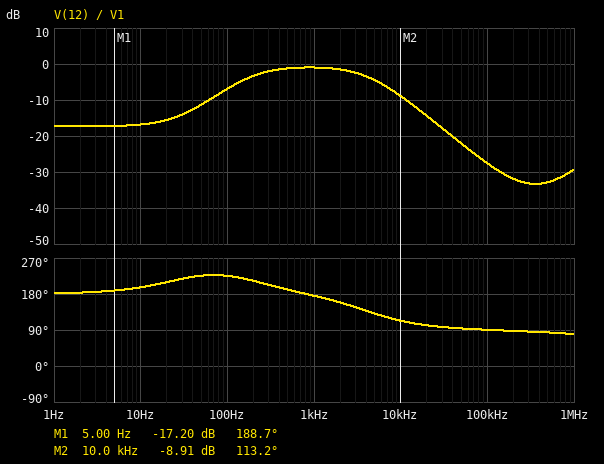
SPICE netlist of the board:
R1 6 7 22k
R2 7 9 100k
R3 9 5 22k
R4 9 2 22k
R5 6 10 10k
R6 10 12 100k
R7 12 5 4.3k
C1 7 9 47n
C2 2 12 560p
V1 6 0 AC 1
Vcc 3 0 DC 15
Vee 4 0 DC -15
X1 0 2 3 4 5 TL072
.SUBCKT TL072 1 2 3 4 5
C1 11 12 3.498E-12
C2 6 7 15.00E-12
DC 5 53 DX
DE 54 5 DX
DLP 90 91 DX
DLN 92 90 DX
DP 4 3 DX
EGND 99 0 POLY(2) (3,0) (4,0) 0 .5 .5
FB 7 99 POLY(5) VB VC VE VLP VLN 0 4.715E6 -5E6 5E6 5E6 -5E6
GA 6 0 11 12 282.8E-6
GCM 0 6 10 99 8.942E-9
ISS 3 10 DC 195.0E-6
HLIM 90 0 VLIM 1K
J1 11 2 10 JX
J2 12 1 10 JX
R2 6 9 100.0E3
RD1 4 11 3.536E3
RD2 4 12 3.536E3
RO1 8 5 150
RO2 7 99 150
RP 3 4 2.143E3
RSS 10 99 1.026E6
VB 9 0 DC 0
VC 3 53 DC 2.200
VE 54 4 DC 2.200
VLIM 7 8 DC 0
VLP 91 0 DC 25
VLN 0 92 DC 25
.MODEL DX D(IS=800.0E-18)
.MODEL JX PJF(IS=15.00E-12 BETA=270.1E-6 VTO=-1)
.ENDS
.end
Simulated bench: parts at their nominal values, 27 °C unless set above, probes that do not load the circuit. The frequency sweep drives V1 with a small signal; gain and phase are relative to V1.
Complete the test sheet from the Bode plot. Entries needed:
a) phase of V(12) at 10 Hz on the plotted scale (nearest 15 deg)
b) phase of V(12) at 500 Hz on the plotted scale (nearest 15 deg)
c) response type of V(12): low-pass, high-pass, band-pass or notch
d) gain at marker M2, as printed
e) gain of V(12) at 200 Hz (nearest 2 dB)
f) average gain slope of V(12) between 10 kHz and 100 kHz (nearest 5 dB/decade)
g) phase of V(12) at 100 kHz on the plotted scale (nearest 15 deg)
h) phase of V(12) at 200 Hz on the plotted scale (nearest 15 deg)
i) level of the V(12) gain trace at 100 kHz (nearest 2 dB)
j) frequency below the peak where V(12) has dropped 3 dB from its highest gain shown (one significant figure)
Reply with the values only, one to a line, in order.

195 deg
195 deg
band-pass
-8.91 dB
-4 dB
-20 dB/decade
90 deg
210 deg
-28 dB
200 Hz
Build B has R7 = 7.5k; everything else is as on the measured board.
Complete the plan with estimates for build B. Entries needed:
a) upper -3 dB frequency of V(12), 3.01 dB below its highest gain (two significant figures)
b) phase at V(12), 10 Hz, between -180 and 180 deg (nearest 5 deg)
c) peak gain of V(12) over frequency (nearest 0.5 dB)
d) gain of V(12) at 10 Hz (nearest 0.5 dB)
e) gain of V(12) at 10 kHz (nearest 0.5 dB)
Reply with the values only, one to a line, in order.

4.4 kHz
-160 deg
-1.5 dB
-19.0 dB
-9.5 dB
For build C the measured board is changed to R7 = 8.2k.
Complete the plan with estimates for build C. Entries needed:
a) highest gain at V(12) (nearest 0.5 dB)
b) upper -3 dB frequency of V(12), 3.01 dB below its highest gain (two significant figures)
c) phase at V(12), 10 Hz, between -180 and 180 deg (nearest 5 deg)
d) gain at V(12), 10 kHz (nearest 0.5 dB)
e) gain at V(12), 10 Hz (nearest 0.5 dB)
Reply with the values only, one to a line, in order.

-1.5 dB
4.4 kHz
-160 deg
-9.5 dB
-19.5 dB
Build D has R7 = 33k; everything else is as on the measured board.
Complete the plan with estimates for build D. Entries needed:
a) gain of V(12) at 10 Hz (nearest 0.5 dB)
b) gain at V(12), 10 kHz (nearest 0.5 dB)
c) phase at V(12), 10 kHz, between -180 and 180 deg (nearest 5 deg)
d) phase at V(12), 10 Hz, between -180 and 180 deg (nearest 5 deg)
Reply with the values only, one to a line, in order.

-20.5 dB
-14.5 dB
110 deg
-20 deg
